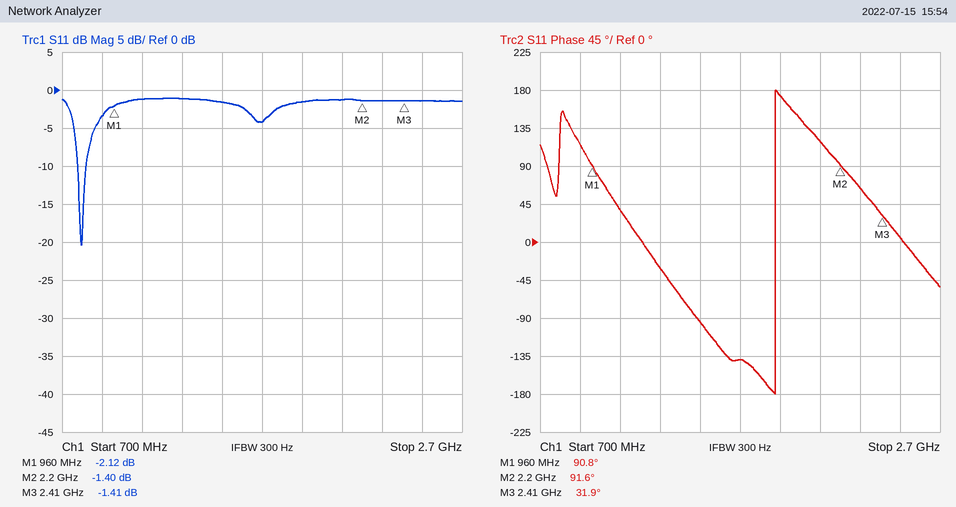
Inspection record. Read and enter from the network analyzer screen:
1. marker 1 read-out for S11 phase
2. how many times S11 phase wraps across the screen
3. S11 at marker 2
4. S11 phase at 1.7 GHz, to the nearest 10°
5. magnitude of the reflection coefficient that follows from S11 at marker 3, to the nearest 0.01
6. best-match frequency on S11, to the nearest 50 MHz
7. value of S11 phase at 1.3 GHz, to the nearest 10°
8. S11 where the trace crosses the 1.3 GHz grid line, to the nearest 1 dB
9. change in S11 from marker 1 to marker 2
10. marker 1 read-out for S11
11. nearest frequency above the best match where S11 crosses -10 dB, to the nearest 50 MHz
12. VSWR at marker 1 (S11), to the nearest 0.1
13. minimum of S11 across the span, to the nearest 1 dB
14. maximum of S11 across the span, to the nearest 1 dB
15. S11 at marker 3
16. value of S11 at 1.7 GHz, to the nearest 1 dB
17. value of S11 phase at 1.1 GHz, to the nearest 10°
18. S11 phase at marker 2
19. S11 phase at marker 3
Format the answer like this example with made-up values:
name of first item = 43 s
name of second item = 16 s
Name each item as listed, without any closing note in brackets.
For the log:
marker 1 read-out for S11 phase = 90.8°
how many times S11 phase wraps across the screen = 1
S11 at marker 2 = -1.40 dB
S11 phase at 1.7 GHz, to the nearest 10° = -140°
magnitude of the reflection coefficient that follows from S11 at marker 3, to the nearest 0.01 = 0.85
best-match frequency on S11, to the nearest 50 MHz = 800 MHz
value of S11 phase at 1.3 GHz, to the nearest 10° = -30°
S11 where the trace crosses the 1.3 GHz grid line, to the nearest 1 dB = -1 dB
change in S11 from marker 1 to marker 2 = 0.72 dB
marker 1 read-out for S11 = -2.12 dB
nearest frequency above the best match where S11 crosses -10 dB, to the nearest 50 MHz = 800 MHz
VSWR at marker 1 (S11), to the nearest 0.1 = 8.2
minimum of S11 across the span, to the nearest 1 dB = -20 dB
maximum of S11 across the span, to the nearest 1 dB = -1 dB
S11 at marker 3 = -1.41 dB
value of S11 at 1.7 GHz, to the nearest 1 dB = -4 dB
value of S11 phase at 1.1 GHz, to the nearest 10° = 40°
S11 phase at marker 2 = 91.6°
S11 phase at marker 3 = 31.9°
